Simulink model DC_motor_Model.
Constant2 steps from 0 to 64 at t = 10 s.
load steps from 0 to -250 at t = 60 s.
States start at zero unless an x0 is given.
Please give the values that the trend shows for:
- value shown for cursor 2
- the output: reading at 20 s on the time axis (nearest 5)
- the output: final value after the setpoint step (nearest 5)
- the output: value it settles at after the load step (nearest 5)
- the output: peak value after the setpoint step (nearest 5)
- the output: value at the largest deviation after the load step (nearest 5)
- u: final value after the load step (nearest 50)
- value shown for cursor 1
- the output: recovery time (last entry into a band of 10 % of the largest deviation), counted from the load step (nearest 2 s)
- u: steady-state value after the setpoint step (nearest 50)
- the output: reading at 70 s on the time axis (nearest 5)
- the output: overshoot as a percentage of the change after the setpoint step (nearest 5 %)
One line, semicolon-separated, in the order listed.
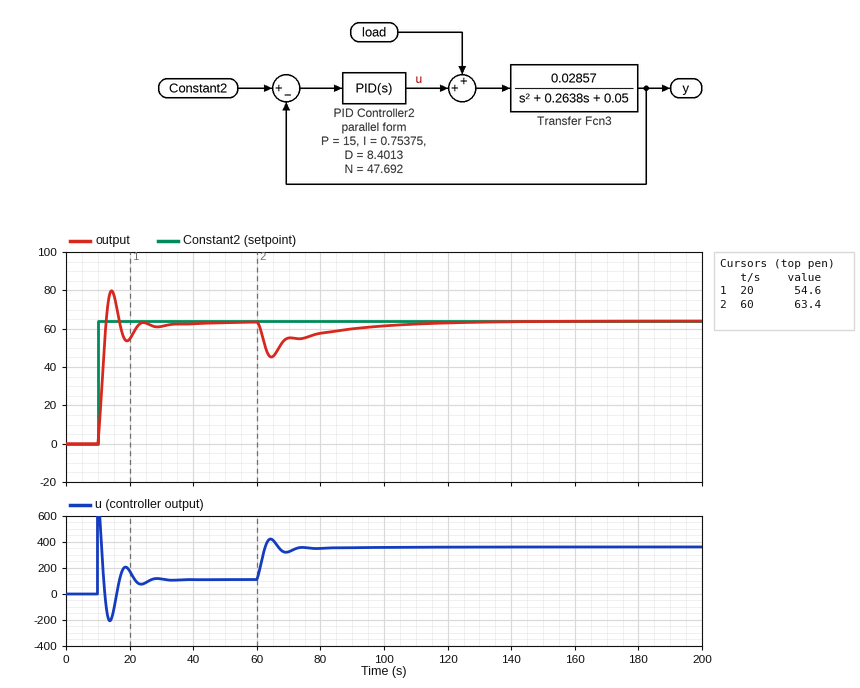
63.4; 55; 65; 65; 80; 45; 350; 54.6; 48 s; 100; 55; 25 %
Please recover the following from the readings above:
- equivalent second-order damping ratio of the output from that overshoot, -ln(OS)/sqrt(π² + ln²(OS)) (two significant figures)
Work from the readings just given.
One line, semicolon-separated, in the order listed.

0.40
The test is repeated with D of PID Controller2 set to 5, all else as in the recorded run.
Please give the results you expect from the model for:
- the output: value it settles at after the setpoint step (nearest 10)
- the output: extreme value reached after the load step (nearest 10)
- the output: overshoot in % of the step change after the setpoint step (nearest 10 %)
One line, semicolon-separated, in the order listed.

60; 40; 30 %
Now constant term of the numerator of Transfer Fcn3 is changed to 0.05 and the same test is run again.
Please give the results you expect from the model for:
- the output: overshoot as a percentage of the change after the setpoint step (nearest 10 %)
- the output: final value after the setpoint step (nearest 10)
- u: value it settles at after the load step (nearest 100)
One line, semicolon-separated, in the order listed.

30 %; 60; 300
